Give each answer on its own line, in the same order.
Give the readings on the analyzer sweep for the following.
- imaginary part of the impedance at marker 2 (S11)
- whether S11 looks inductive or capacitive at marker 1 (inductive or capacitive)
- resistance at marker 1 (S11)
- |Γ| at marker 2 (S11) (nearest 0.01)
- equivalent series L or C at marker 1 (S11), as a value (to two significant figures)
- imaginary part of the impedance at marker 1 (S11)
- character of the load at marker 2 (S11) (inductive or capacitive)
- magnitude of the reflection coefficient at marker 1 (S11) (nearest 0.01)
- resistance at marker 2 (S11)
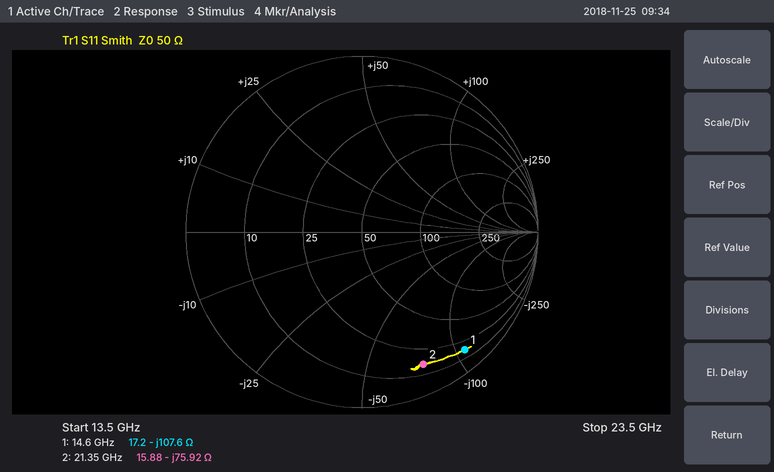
-75.92 Ω
capacitive
17.2 Ω
0.83
100 fF
-107.6 Ω
capacitive
0.89
15.88 Ω
